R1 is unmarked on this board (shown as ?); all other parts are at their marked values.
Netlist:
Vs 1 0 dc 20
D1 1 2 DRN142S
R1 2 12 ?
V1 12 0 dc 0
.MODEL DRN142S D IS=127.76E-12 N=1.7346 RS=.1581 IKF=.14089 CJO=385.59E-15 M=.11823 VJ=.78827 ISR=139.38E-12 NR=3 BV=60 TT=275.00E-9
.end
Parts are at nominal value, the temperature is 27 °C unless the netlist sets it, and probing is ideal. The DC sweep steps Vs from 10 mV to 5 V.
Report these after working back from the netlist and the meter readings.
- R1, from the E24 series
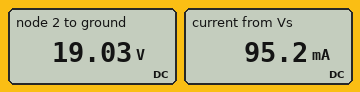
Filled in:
200 Ω
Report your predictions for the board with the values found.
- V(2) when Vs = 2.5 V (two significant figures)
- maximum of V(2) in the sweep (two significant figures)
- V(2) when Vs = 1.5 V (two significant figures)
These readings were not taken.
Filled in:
1.7 V
4.1 V
720 mV
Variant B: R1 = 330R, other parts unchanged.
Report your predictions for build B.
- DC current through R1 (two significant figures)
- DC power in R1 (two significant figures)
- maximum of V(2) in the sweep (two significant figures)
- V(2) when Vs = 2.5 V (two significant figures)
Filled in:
58 mA
1.1 W
4.2 V
1.7 V
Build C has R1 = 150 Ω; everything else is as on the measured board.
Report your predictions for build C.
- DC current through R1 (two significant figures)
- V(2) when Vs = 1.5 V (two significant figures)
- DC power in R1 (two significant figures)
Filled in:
130 mA
710 mV
2.4 W
